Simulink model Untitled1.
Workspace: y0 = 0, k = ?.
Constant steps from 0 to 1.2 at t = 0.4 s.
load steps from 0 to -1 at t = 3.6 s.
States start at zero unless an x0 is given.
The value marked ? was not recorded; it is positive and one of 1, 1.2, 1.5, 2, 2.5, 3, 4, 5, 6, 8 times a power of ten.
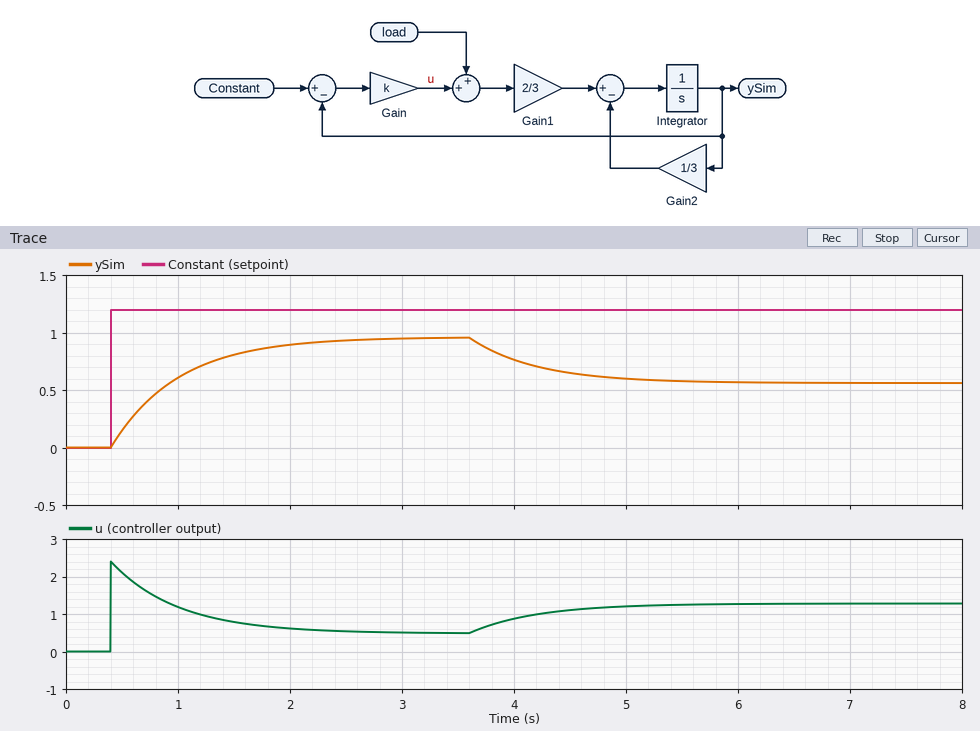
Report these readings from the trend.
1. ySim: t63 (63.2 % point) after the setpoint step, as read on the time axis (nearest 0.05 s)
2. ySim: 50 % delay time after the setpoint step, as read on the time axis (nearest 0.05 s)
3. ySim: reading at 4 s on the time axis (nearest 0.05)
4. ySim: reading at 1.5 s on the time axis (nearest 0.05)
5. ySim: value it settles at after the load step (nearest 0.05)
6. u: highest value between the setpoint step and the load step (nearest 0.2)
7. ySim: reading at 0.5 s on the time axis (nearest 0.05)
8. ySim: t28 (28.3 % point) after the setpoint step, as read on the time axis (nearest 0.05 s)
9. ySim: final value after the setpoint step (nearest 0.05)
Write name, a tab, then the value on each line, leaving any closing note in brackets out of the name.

ySim: t63 (63.2 % point) after the setpoint step, as read on the time axis	1.00 s
ySim: 50 % delay time after the setpoint step, as read on the time axis	0.80 s
ySim: reading at 4 s on the time axis	0.75
ySim: reading at 1.5 s on the time axis	0.80
ySim: value it settles at after the load step	0.55
u: highest value between the setpoint step and the load step	2.4
ySim: reading at 0.5 s on the time axis	0.15
ySim: t28 (28.3 % point) after the setpoint step, as read on the time axis	0.60 s
ySim: final value after the setpoint step	0.95
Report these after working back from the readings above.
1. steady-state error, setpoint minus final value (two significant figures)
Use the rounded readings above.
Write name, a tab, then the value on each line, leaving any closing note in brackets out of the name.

steady-state error, setpoint minus final value	0.25
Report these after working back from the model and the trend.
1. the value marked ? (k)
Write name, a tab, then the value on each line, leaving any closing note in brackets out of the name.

the value marked ?	2
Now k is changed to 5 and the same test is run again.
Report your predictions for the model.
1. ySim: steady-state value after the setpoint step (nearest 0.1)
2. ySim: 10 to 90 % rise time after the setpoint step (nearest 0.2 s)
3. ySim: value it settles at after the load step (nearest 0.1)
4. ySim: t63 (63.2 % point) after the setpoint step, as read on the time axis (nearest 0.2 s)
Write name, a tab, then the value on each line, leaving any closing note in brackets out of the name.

ySim: steady-state value after the setpoint step	1.1
ySim: 10 to 90 % rise time after the setpoint step	0.6 s
ySim: value it settles at after the load step	0.9
ySim: t63 (63.2 % point) after the setpoint step, as read on the time axis	0.6 s
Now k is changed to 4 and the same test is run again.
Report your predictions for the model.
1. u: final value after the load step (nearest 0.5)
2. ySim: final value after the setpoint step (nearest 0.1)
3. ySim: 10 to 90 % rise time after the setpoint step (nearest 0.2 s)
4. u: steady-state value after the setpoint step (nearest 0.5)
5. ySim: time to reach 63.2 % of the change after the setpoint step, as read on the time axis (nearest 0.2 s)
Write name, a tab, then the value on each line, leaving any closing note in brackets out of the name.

u: final value after the load step	1.5
ySim: final value after the setpoint step	1.1
ySim: 10 to 90 % rise time after the setpoint step	0.8 s
u: steady-state value after the setpoint step	0.5
ySim: time to reach 63.2 % of the change after the setpoint step, as read on the time axis	0.8 s
